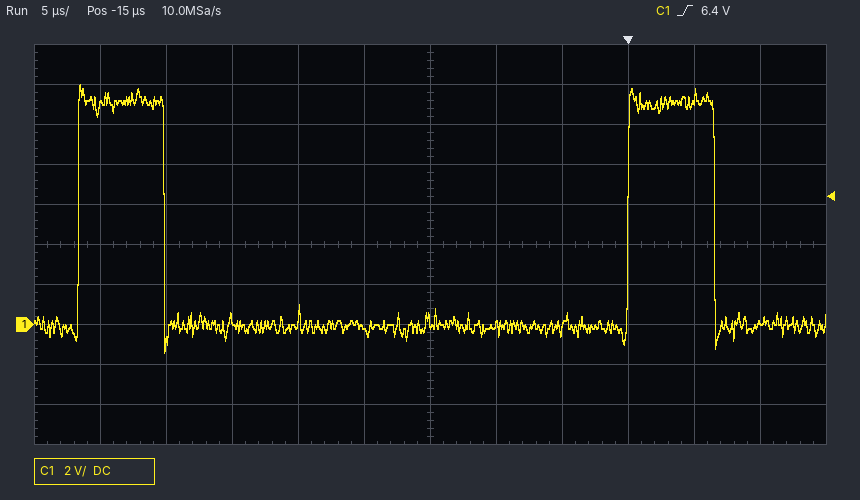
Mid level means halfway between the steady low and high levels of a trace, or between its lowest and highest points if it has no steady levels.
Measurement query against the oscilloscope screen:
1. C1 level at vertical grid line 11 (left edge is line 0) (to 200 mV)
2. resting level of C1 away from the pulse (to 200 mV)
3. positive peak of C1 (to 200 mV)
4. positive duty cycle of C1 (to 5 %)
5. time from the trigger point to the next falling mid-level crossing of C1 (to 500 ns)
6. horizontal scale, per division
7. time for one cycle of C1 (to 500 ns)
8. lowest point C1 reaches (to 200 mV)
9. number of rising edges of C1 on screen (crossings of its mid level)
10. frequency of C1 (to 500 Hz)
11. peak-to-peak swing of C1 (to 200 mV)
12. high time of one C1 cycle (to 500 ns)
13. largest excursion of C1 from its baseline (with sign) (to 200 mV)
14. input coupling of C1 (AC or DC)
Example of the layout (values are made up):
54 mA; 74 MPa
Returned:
0.0 V; 0.0 V; 12.0 V; 15 %; 6.5 µs; 5 µs; 41.5 µs; -1.4 V; 2; 24.0 kHz; 13.4 V; 6.5 µs; +12.0 V; DC
